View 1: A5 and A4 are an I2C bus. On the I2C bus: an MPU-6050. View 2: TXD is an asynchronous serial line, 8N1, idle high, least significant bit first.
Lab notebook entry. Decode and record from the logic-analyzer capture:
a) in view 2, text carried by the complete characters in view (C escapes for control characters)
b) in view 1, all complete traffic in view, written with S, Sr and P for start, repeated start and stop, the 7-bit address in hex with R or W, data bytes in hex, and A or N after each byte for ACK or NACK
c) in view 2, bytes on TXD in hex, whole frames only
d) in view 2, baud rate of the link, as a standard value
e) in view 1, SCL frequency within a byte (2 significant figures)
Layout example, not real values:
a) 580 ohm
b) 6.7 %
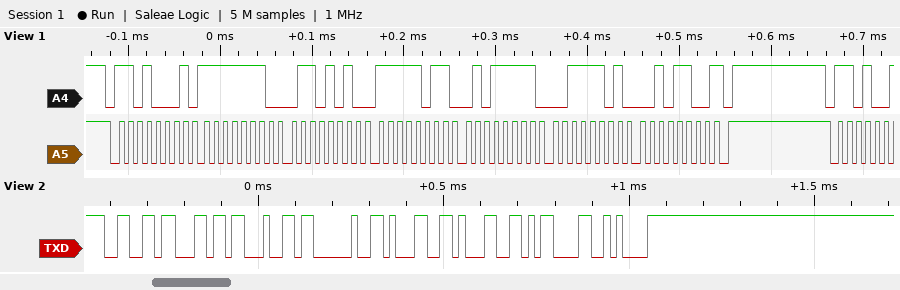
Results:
a) "fld 11\r\n"
b) S 68R A FE A 6A A FB A 5F A 3D A 2C N P
c) 66 6C 64 20 31 31 0D 0A
d) 57600 baud
e) 100 kHz
